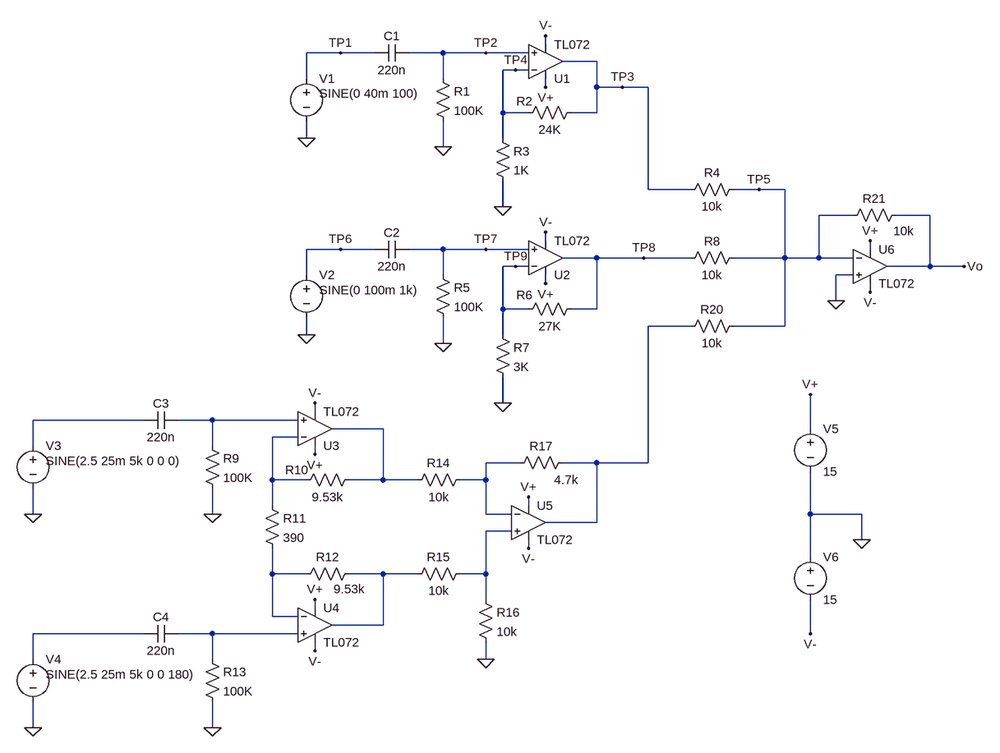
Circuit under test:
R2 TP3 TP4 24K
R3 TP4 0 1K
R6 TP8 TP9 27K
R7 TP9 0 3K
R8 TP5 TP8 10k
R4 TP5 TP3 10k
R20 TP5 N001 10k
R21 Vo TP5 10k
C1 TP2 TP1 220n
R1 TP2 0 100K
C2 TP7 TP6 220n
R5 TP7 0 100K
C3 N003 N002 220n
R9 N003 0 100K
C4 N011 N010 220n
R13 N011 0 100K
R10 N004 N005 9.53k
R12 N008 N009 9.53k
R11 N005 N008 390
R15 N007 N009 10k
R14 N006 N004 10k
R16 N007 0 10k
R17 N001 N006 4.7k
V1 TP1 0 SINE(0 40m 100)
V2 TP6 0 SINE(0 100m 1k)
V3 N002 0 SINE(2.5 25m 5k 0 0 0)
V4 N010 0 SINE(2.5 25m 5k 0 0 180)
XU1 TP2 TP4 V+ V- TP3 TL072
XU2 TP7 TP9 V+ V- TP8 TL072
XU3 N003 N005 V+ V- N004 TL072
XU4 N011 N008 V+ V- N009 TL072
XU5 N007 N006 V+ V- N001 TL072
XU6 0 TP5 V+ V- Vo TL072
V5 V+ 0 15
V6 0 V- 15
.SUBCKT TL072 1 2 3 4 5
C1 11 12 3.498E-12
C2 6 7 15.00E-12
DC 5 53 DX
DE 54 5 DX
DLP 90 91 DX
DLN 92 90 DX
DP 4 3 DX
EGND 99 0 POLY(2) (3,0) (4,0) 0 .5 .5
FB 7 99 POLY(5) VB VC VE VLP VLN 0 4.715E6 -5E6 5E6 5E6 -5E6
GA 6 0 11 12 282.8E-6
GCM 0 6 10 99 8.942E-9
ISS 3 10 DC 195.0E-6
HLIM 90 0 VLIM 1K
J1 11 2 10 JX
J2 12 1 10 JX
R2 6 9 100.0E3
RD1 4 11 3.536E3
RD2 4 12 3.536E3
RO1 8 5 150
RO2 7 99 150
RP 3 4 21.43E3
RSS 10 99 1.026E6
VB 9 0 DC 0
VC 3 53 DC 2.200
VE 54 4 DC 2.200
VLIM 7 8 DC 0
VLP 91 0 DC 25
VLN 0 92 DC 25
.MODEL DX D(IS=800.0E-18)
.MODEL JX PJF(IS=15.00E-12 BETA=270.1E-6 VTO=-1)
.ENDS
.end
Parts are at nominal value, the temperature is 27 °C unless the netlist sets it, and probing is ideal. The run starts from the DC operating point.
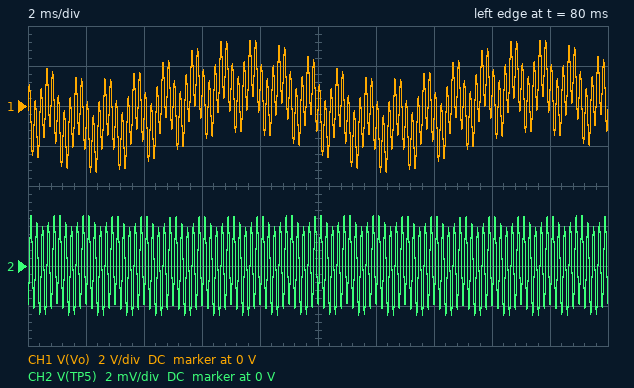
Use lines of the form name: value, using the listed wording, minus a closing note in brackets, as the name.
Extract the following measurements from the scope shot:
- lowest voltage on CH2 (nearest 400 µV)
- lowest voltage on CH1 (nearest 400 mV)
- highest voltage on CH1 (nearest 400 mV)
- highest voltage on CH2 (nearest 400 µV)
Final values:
lowest voltage on CH2: -2.4 mV
lowest voltage on CH1: -3.2 V
highest voltage on CH1: 3.2 V
highest voltage on CH2: 2.4 mV
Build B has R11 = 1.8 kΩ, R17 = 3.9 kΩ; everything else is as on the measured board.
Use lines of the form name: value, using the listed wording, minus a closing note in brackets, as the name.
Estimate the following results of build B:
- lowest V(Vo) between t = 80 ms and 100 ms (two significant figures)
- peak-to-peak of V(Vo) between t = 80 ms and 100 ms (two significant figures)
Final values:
lowest V(Vo) between t = 80 ms and 100 ms: -2.1 V
peak-to-peak of V(Vo) between t = 80 ms and 100 ms: 4.3 V
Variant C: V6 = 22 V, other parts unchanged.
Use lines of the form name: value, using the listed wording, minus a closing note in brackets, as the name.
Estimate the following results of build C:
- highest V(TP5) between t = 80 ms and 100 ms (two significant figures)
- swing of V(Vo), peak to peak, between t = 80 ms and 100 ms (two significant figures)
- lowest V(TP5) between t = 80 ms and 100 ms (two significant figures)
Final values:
highest V(TP5) between t = 80 ms and 100 ms: 2.4 mV
swing of V(Vo), peak to peak, between t = 80 ms and 100 ms: 6.6 V
lowest V(TP5) between t = 80 ms and 100 ms: -2.6 mV
